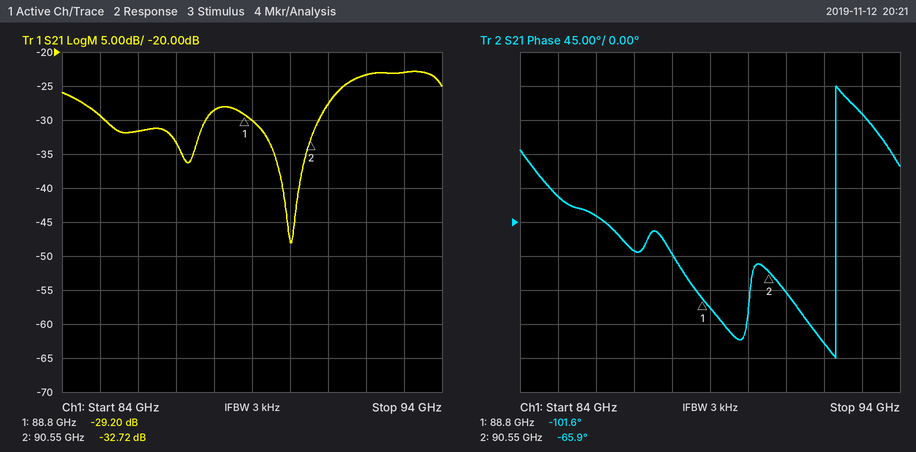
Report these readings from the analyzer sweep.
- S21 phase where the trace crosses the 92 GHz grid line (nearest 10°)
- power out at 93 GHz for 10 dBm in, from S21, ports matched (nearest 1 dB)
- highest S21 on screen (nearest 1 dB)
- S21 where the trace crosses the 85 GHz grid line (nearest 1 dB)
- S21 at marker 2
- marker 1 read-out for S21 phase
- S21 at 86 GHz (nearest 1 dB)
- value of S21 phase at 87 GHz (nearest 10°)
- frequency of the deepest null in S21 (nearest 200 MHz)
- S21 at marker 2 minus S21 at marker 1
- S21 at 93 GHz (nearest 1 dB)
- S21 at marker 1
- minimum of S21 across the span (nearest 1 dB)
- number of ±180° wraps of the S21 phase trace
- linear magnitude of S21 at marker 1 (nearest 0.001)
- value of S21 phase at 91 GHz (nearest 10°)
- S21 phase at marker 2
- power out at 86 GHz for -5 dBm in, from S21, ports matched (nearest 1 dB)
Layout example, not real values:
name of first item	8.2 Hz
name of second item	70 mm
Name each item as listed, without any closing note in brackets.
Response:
S21 phase where the trace crosses the 92 GHz grid line	-160°
power out at 93 GHz for 10 dBm in, from S21, ports matched	-13 dBm
highest S21 on screen	-23 dB
S21 where the trace crosses the 85 GHz grid line	-29 dB
S21 at marker 2	-32.72 dB
marker 1 read-out for S21 phase	-101.6°
S21 at 86 GHz	-32 dB
value of S21 phase at 87 GHz	-40°
frequency of the deepest null in S21	90.0 GHz
S21 at marker 2 minus S21 at marker 1	-3.52 dB
S21 at 93 GHz	-23 dB
S21 at marker 1	-29.20 dB
minimum of S21 across the span	-48 dB
number of ±180° wraps of the S21 phase trace	1
linear magnitude of S21 at marker 1	0.035
value of S21 phase at 91 GHz	-90°
S21 phase at marker 2	-65.9°
power out at 86 GHz for -5 dBm in, from S21, ports matched	-37 dBm
